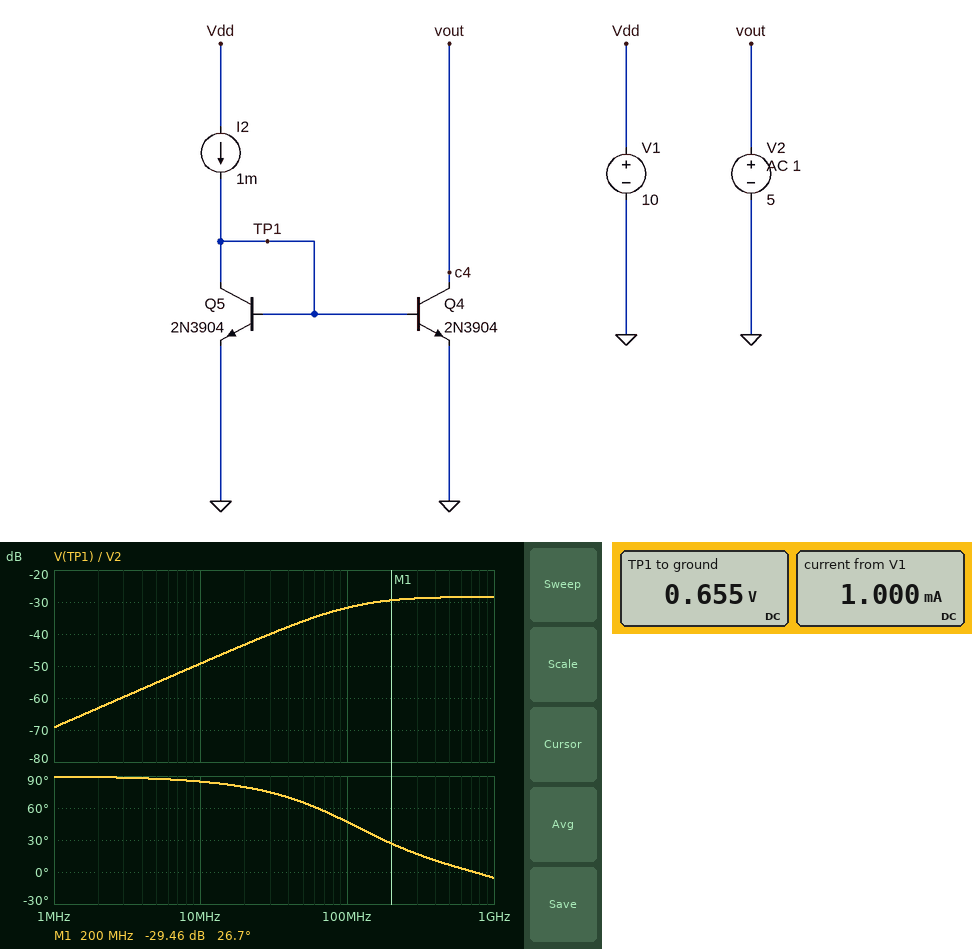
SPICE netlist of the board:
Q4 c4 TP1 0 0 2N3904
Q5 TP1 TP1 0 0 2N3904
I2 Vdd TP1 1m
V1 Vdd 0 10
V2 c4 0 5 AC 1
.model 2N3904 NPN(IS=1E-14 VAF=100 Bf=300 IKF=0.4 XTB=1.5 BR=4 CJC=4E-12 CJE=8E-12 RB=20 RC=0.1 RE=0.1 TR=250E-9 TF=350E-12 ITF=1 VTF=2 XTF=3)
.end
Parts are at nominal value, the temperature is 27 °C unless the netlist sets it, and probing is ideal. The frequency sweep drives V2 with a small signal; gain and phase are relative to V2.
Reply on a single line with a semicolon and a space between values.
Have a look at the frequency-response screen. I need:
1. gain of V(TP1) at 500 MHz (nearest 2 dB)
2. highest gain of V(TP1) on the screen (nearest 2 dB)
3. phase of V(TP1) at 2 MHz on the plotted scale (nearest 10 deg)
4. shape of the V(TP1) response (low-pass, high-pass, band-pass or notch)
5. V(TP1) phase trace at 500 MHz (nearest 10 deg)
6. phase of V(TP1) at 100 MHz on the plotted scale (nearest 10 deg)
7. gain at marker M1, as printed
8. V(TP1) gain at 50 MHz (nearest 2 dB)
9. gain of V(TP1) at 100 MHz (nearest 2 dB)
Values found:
-28 dB; -28 dB; 90 deg; high-pass; 10 deg; 50 deg; -29.46 dB; -36 dB; -32 dB
